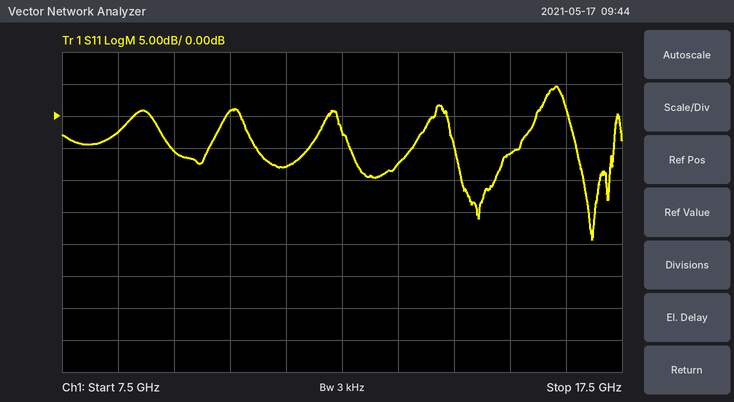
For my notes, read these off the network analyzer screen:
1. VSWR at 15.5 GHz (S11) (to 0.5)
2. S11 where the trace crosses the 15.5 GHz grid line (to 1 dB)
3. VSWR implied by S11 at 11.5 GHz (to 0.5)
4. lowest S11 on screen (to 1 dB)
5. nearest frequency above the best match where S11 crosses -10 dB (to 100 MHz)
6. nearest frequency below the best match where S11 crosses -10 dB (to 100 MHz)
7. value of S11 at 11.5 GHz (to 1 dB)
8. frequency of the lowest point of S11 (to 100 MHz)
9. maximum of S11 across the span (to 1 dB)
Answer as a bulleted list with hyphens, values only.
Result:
- 3.0
- -6 dB
- 2.5
- -19 dB
- 17.1 GHz
- 16.8 GHz
- -8 dB
- 17.0 GHz
- 5 dB
